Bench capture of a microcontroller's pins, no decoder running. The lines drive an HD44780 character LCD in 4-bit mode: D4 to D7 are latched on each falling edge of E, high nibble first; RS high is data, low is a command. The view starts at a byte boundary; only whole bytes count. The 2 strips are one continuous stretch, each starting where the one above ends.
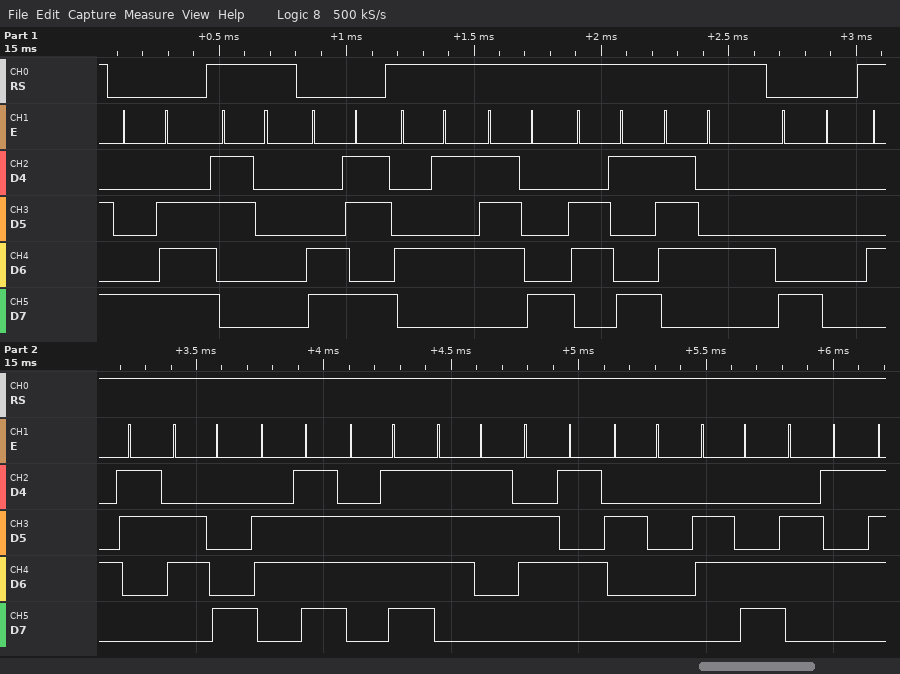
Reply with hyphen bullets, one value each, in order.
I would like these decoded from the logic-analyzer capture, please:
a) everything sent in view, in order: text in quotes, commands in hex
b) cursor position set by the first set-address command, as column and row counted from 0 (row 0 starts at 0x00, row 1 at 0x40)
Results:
- 0x8E "0" 0xCB "Exit" 0x80 "Choose le"
- column 14, row 0
